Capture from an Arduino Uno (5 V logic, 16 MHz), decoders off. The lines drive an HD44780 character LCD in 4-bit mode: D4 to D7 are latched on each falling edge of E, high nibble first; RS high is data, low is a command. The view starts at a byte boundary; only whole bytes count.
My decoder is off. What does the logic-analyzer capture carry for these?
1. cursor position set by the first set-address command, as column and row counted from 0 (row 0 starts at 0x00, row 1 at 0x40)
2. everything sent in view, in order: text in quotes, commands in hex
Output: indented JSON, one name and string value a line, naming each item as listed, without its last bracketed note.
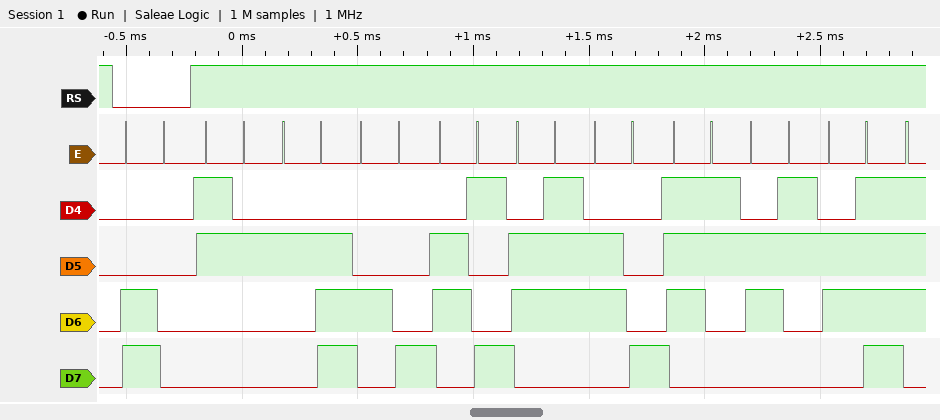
{
  "cursor position set by the first set-address command, as column and row counted from 0": "column 0, row 1",
  "everything sent in view, in order: text in quotes, commands in hex": "0xC0 \"2.Highsco\""
}
